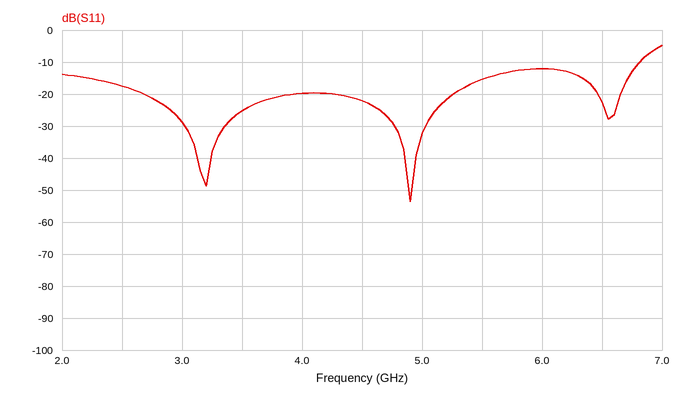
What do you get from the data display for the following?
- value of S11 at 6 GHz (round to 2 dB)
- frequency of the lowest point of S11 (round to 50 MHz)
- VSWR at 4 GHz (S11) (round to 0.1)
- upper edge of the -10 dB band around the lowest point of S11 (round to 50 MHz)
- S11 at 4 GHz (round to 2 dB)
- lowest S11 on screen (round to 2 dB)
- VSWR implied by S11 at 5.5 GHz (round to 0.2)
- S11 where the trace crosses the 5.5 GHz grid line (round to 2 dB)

-12 dB
4.90 GHz
1.2
6.80 GHz
-20 dB
-54 dB
1.4
-16 dB
